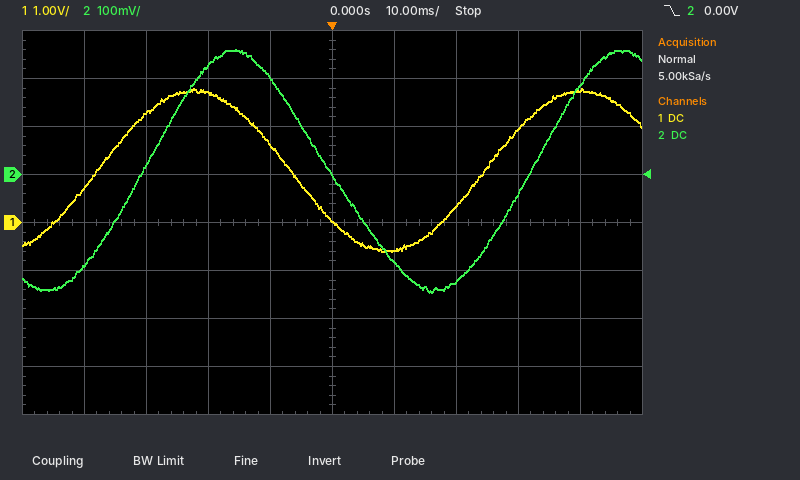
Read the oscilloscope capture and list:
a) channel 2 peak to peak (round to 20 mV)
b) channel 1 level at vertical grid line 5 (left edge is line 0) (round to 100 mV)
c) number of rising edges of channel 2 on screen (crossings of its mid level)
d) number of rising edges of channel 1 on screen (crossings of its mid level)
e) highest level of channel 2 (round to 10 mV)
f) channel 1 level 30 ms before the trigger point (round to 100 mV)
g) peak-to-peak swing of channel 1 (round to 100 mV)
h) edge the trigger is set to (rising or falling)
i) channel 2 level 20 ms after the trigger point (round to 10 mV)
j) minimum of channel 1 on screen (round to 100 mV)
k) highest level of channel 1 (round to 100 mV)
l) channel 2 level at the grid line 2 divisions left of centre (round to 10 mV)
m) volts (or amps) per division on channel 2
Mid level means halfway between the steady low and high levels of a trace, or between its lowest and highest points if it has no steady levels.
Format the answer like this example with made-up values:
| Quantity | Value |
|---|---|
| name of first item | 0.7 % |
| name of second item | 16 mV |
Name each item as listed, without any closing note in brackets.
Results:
| Quantity | Value |
|---|---|
| channel 2 peak to peak | 500 mV |
| channel 1 level at vertical grid line 5 (left edge is line 0) | 0.0 V |
| number of rising edges of channel 2 on screen | 2 |
| number of rising edges of channel 1 on screen | 2 |
| highest level of channel 2 | 260 mV |
| channel 1 level 30 ms before the trigger point | 2.3 V |
| peak-to-peak swing of channel 1 | 3.4 V |
| edge the trigger is set to | falling |
| channel 2 level 20 ms after the trigger point | -220 mV |
| minimum of channel 1 on screen | -600 mV |
| highest level of channel 1 | 2.8 V |
| channel 2 level at the grid line 2 divisions left of centre | 230 mV |
| volts (or amps) per division on channel 2 | 100 mV |
